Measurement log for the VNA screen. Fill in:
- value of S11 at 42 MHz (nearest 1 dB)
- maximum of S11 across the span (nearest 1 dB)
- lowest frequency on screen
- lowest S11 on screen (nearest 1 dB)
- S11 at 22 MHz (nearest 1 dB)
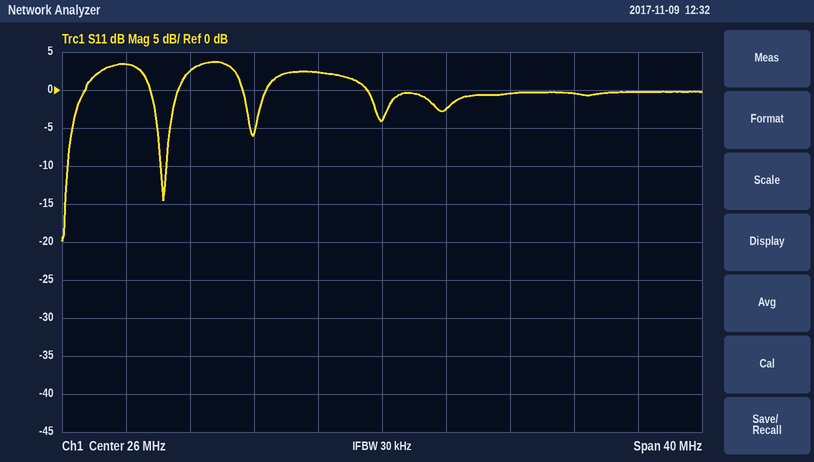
0 dB
4 dB
6 MHz
-20 dB
2 dB
